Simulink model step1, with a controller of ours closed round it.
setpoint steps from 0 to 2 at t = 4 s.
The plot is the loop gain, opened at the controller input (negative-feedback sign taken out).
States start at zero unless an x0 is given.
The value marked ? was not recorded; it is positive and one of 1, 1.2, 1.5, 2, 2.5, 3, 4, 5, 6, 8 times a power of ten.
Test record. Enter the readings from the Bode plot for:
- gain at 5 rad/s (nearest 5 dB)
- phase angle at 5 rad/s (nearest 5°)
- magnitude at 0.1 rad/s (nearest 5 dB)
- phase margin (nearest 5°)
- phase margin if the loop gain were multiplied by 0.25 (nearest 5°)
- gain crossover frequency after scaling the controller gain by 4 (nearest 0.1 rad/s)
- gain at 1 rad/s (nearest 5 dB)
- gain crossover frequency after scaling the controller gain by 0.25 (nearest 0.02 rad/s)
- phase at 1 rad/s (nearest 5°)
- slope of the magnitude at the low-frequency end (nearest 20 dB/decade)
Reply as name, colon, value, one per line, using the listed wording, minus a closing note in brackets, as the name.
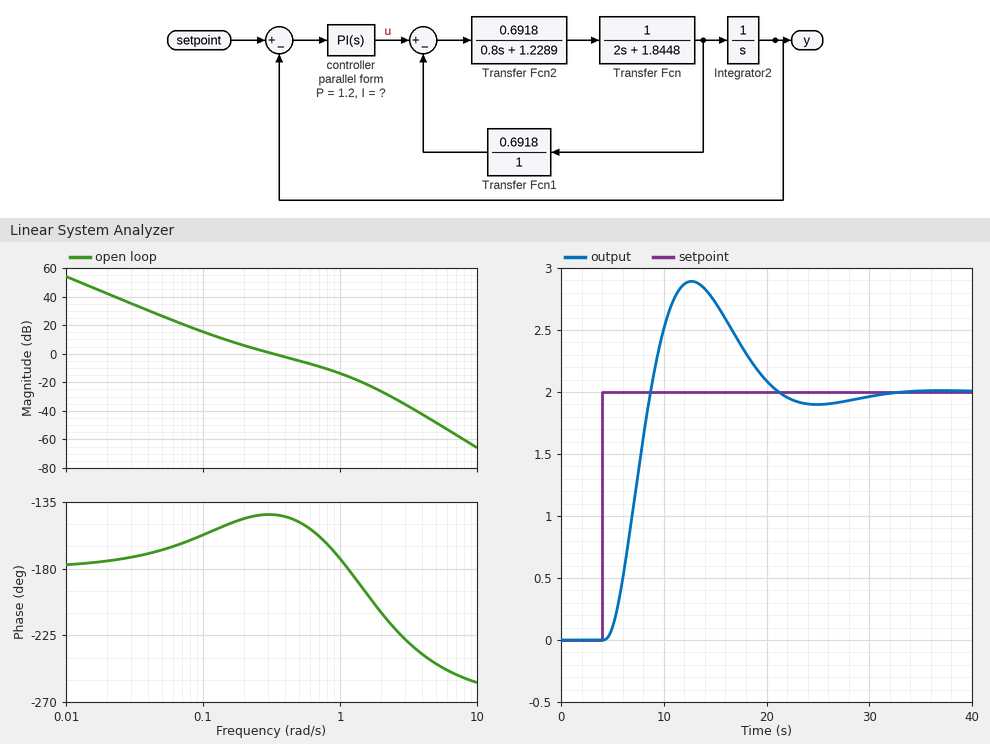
gain at 5 rad/s: -50 dB
phase angle at 5 rad/s: -245°
magnitude at 0.1 rad/s: 15 dB
phase margin: 35°
phase margin if the loop gain were multiplied by 0.25: 25°
gain crossover frequency after scaling the controller gain by 4: 0.9 rad/s
gain at 1 rad/s: -15 dB
gain crossover frequency after scaling the controller gain by 0.25: 0.12 rad/s
phase at 1 rad/s: -175°
slope of the magnitude at the low-frequency end: -40 dB/decade
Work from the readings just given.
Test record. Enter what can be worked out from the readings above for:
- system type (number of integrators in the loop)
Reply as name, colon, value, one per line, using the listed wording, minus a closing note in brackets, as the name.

system type: 2
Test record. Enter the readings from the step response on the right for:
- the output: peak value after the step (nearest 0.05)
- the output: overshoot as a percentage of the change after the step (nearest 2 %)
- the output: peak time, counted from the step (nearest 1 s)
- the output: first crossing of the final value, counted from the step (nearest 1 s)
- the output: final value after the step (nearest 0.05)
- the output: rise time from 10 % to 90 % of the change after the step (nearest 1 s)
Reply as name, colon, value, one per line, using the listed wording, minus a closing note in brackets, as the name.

the output: peak value after the step: 2.90
the output: overshoot as a percentage of the change after the step: 44 %
the output: peak time, counted from the step: 9 s
the output: first crossing of the final value, counted from the step: 5 s
the output: final value after the step: 2.00
the output: rise time from 10 % to 90 % of the change after the step: 3 s
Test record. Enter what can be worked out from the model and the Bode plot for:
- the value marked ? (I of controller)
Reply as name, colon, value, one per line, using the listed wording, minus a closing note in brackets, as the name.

the value marked ?: 0.2
